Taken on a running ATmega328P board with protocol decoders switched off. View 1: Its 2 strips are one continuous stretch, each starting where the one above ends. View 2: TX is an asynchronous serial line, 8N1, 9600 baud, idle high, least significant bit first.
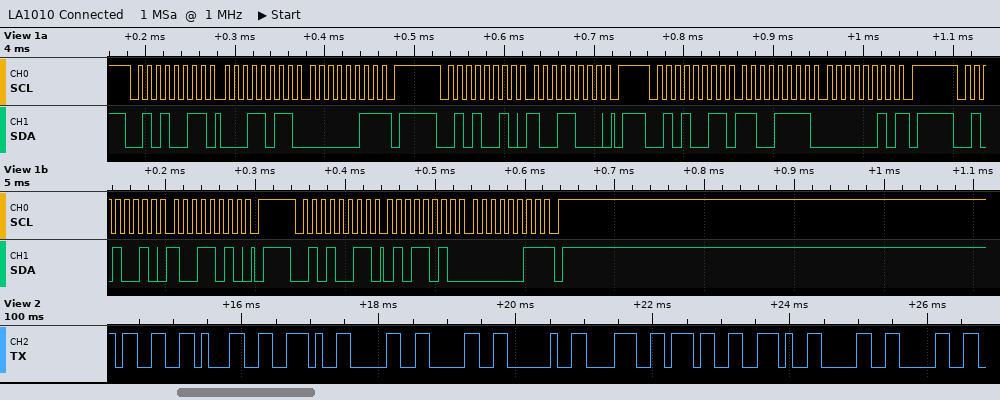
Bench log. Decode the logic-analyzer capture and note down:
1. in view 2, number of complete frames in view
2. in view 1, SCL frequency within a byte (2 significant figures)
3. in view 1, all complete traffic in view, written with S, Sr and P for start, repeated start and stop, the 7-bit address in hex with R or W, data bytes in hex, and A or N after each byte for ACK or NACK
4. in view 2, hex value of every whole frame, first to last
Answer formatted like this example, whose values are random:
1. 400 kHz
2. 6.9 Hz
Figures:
1. 11
2. 100 kHz
3. S 29R A 1B A 03 N P S 29W A 98 A P S 29R A CF A 02 N P S 29W A 9A A P S 29R A 5A A 03 N P
4. 33 31 2E 30 30 20 38 37 2E 30 30
